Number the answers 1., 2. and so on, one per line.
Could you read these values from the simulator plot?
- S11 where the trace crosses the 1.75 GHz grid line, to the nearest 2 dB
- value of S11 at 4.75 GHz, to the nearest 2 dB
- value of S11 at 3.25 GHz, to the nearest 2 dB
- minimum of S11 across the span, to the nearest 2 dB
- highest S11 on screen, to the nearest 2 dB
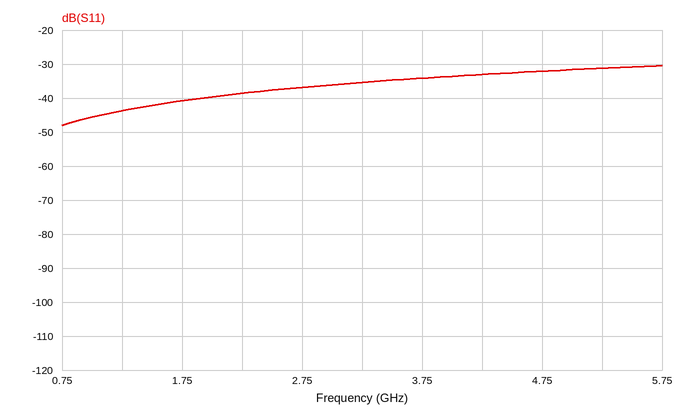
1. -40 dB
2. -32 dB
3. -36 dB
4. -48 dB
5. -30 dB
